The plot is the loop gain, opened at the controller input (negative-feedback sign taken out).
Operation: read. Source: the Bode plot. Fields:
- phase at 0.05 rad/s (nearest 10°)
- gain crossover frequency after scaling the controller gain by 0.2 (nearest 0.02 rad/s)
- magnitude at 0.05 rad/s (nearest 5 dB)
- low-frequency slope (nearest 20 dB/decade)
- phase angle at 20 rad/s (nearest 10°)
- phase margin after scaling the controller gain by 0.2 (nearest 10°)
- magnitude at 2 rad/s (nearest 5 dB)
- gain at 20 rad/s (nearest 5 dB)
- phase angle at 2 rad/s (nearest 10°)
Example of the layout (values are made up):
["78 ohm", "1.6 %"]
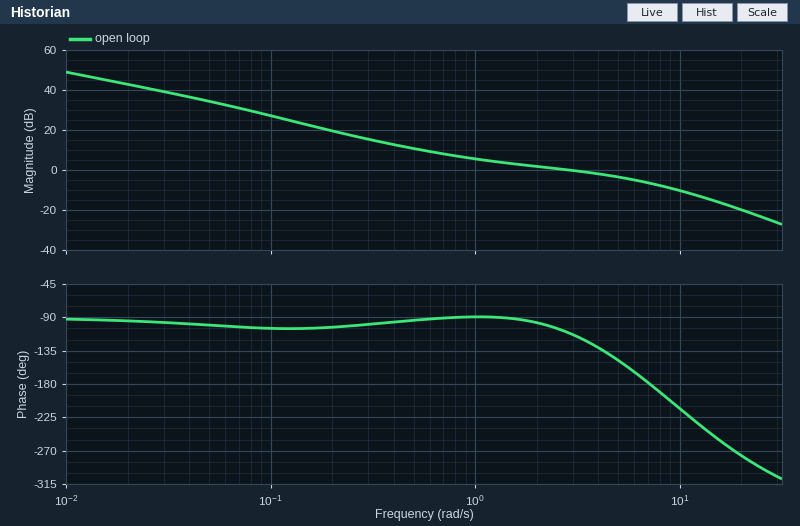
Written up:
["-100°", "0.34 rad/s", "35 dB", "-20 dB/decade", "-280°", "80°", "0 dB", "-20 dB", "-100°"]
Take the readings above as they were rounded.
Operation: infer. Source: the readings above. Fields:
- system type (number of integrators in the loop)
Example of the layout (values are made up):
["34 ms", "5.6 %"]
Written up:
["1"]
